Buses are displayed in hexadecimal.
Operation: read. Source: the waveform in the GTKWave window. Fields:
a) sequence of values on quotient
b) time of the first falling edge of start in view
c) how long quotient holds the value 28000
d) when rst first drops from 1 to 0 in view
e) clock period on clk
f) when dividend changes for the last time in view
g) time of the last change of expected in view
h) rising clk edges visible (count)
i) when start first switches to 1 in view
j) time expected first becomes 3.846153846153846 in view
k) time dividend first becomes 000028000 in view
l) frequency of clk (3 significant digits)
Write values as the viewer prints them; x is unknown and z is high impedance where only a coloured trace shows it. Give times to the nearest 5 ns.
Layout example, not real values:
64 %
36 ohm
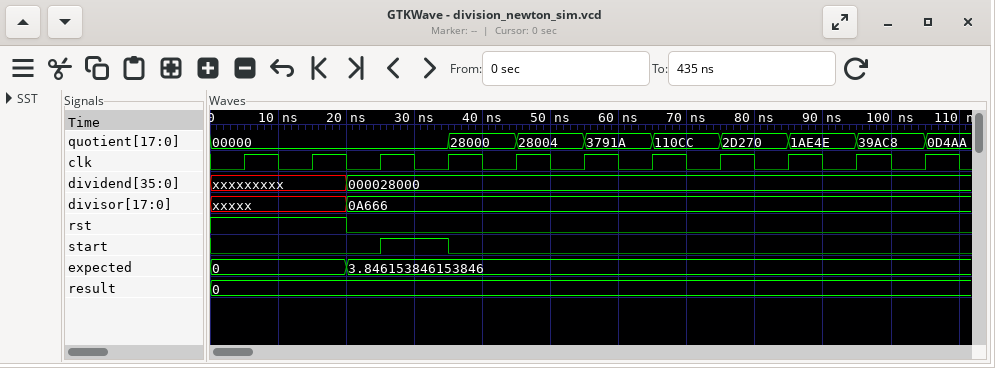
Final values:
00000, 28000, 28004, 3791A, 110CC, 2D270, 1AE4E, 39AC8, 0D4AA
35 ns
10 ns
20 ns
10 ns
20 ns
20 ns
11
25 ns
20 ns
20 ns
100 MHz
